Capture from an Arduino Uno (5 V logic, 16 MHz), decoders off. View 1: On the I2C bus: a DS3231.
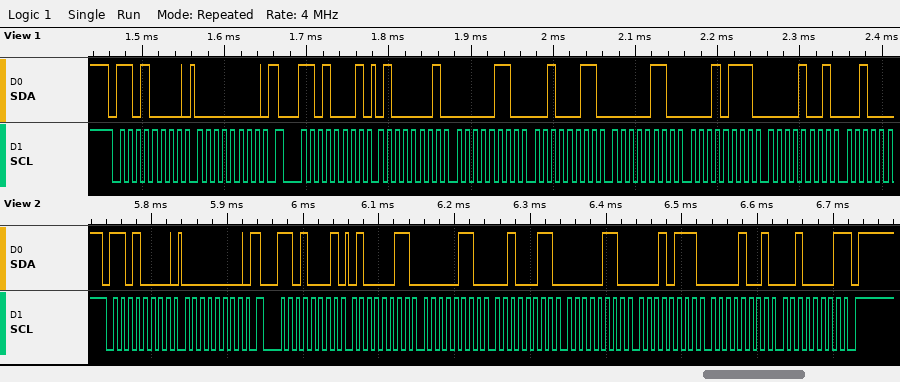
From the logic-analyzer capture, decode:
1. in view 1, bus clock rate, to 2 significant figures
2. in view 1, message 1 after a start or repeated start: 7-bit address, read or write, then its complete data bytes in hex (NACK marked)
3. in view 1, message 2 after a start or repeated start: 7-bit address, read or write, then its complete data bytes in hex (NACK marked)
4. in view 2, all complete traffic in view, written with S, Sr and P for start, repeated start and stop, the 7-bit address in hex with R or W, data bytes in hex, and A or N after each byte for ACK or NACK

100 kHz
0x68 write: 00
0x68 read: 41 06 23 06 17 09
S 68W A 00 A Sr 68R A 43 A 06 A 23 A 06 A 17 A 09 A 21 N P
